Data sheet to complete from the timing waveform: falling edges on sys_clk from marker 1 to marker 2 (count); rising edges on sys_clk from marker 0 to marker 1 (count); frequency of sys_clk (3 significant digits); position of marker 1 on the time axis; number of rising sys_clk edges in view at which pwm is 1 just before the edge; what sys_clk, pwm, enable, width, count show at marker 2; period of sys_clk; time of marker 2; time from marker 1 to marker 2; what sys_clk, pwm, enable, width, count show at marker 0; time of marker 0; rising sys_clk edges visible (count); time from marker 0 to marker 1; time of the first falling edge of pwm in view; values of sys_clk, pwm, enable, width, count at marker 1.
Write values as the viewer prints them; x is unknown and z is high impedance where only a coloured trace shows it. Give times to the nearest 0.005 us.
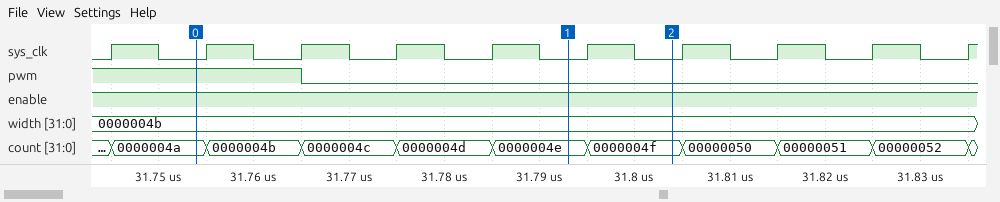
1
4
100 MHz
31.795 us
3
sys_clk=0, pwm=0, enable=1, width=0000004b, count=0000004f
0.01 us
31.805 us
0.01 us
sys_clk=0, pwm=1, enable=1, width=0000004b, count=0000004a
31.755 us
10
0.04 us
31.765 us
sys_clk=0, pwm=0, enable=1, width=0000004b, count=0000004e
